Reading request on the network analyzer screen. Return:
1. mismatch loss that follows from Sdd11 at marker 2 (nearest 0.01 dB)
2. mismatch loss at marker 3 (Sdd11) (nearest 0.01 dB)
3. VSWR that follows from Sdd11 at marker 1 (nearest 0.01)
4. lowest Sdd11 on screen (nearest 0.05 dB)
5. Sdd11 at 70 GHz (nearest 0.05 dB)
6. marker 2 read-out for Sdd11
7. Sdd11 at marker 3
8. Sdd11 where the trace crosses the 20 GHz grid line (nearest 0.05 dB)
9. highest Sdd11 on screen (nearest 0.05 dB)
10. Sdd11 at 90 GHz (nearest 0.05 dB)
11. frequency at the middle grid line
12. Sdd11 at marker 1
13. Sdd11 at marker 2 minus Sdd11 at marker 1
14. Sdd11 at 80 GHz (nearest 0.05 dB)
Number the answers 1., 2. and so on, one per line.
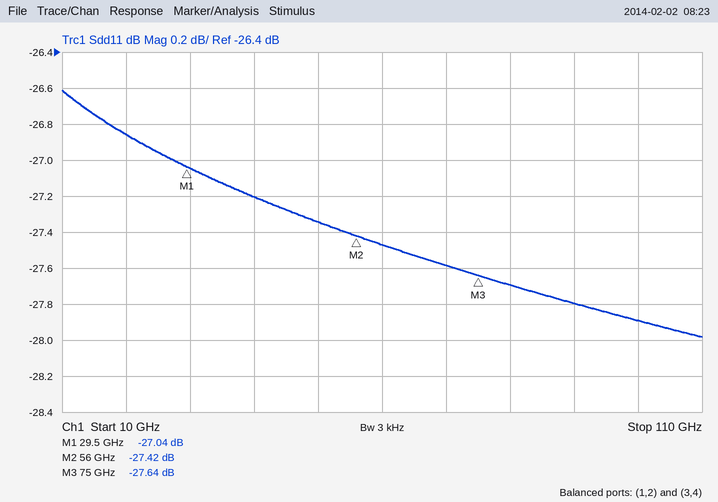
1. 0.01 dB
2. 0.01 dB
3. 1.09
4. -28.00 dB
5. -27.60 dB
6. -27.42 dB
7. -27.64 dB
8. -26.85 dB
9. -26.60 dB
10. -27.80 dB
11. 60 GHz
12. -27.04 dB
13. -0.38 dB
14. -27.70 dB
